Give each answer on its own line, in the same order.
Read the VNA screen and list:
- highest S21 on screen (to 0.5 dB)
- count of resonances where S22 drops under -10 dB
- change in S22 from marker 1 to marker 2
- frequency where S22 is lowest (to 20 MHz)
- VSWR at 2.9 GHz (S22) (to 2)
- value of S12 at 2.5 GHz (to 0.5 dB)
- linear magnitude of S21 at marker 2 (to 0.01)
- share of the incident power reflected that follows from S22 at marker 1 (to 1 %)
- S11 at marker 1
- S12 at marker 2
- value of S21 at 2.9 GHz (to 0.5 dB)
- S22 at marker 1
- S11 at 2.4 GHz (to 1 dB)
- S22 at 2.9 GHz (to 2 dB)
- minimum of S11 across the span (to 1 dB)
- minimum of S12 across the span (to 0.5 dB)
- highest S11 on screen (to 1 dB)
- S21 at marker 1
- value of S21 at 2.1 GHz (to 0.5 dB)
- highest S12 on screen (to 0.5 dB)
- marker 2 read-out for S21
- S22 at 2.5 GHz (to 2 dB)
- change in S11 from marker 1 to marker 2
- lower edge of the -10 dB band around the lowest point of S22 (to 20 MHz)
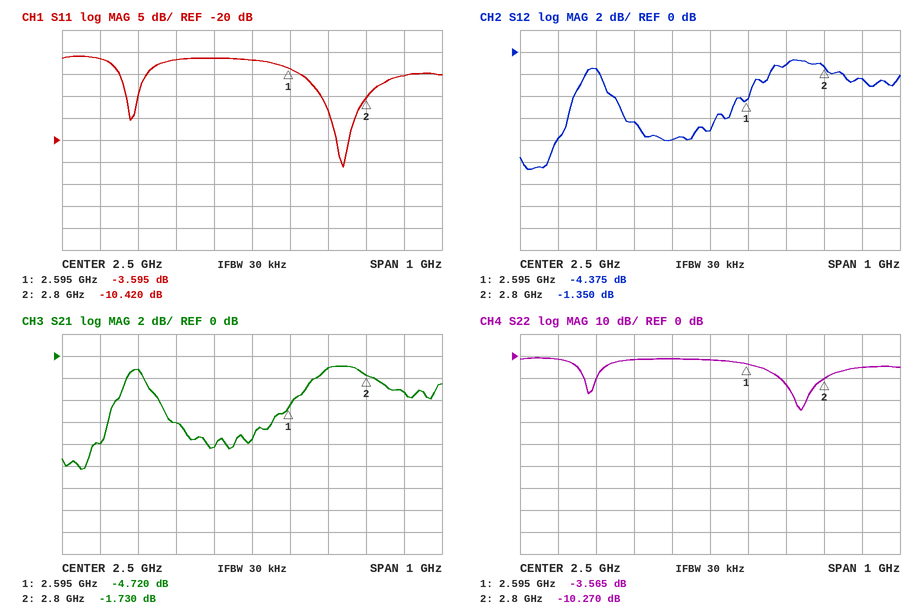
-1.0 dB
2
-6.705 dB
2.74 GHz
4
-7.0 dB
0.82
44 %
-3.595 dB
-1.350 dB
-3.5 dB
-3.565 dB
-1 dB
-6 dB
-26 dB
-10.5 dB
-1 dB
-4.720 dB
-8.0 dB
-0.5 dB
-1.730 dB
-2 dB
-6.825 dB
2.68 GHz
